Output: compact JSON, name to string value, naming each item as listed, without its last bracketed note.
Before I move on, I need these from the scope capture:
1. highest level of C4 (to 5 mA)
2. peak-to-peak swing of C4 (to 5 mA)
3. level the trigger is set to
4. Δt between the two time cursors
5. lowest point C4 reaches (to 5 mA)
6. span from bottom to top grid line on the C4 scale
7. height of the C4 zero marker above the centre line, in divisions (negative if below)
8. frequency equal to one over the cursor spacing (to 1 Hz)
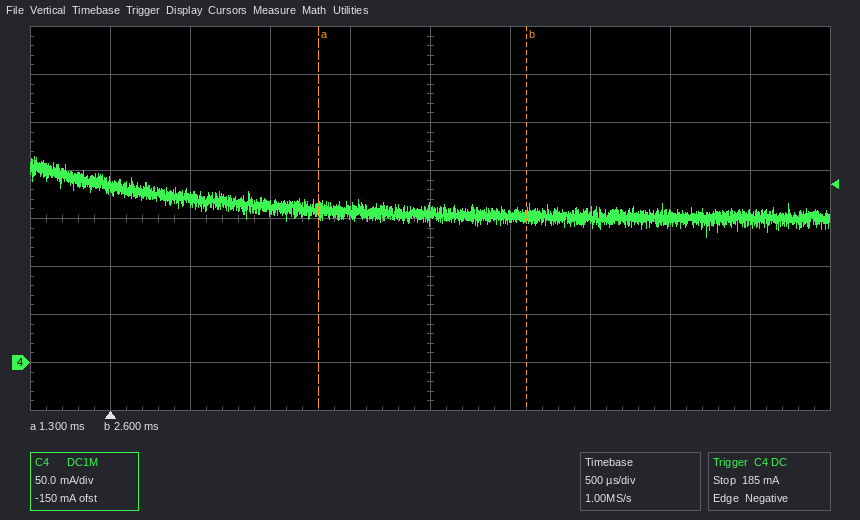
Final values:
{"highest level of C4": "215 mA", "peak-to-peak swing of C4": "85 mA", "level the trigger is set to": "185 mA", "Δt between the two time cursors": "1.30 ms", "lowest point C4 reaches": "130 mA", "span from bottom to top grid line on the C4 scale": "400 mA", "height of the C4 zero marker above the centre line, in divisions": "-3.0 div", "frequency equal to one over the cursor spacing": "769 Hz"}
